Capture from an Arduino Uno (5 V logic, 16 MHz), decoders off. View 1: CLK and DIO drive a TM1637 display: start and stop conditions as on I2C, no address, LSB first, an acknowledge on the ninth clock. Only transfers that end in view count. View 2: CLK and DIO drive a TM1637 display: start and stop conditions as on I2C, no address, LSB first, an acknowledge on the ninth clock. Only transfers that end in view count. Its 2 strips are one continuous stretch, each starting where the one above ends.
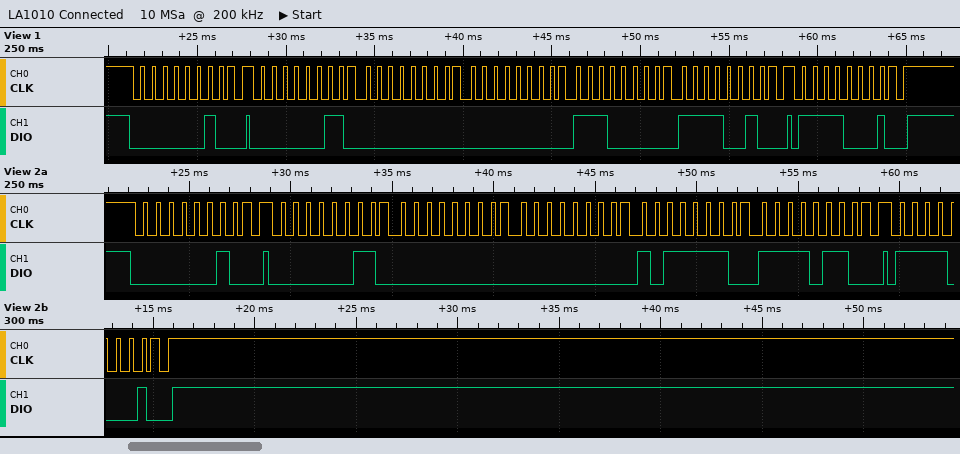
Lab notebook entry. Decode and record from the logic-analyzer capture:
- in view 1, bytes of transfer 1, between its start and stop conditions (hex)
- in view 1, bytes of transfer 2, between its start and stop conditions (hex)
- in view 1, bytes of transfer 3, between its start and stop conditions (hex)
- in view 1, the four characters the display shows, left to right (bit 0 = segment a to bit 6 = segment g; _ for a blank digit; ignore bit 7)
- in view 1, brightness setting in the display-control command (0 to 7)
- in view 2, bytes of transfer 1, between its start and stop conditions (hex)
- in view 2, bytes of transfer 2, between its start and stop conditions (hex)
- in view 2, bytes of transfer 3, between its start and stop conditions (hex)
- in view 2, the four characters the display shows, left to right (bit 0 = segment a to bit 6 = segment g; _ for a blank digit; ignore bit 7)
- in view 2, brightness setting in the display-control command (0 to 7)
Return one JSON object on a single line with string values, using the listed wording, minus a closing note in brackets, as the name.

{"in view 1, bytes of transfer 1, between its start and stop conditions": "40", "in view 1, bytes of transfer 2, between its start and stop conditions": "C0 00 00 07 4F", "in view 1, bytes of transfer 3, between its start and stop conditions": "8F", "in view 1, the four characters the display shows, left to right": "__73", "in view 1, brightness setting in the display-control command": "7", "in view 2, bytes of transfer 1, between its start and stop conditions": "40", "in view 2, bytes of transfer 2, between its start and stop conditions": "C0 00 00 7D 6F", "in view 2, bytes of transfer 3, between its start and stop conditions": "8F", "in view 2, the four characters the display shows, left to right": "__69", "in view 2, brightness setting in the display-control command": "7"}
